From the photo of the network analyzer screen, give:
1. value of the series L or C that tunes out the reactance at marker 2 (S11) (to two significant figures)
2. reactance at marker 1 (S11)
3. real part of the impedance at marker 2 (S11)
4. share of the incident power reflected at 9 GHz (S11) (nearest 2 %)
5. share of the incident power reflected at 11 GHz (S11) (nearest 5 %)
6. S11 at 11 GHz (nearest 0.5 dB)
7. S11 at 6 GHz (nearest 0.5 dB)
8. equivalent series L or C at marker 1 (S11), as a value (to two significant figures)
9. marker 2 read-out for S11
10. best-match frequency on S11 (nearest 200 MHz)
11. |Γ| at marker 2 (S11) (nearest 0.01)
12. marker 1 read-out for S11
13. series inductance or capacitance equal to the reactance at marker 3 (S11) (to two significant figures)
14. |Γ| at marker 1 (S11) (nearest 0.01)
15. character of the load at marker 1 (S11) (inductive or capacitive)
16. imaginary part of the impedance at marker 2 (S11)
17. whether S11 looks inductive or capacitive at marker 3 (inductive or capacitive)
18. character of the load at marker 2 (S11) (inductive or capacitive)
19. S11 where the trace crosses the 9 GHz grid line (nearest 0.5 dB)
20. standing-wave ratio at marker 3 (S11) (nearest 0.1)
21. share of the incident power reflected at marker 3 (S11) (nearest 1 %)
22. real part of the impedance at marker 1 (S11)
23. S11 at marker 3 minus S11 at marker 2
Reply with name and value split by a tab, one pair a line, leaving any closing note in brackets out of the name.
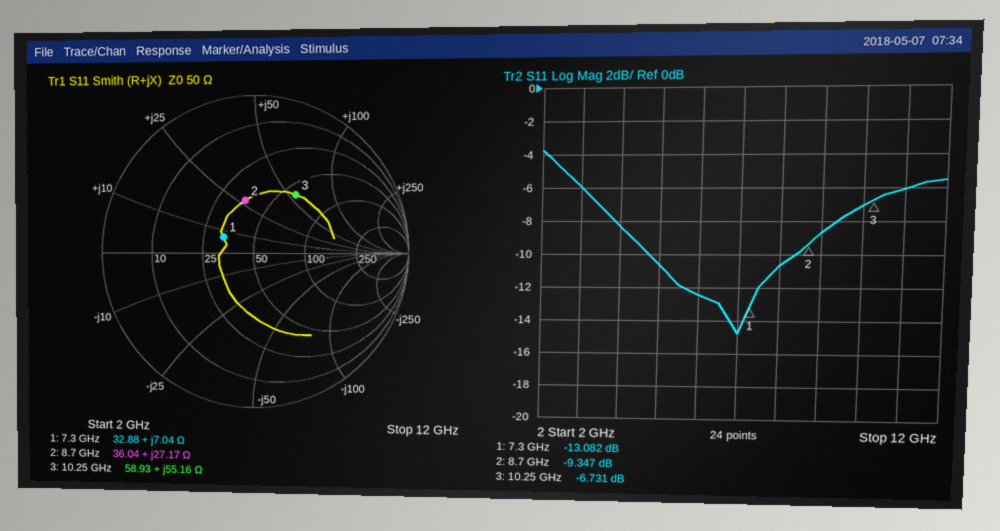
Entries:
value of the series L or C that tunes out the reactance at marker 2 (S11)	670 fF
reactance at marker 1	+7.04 Ω
real part of the impedance at marker 2	36.04 Ω
share of the incident power reflected at 9 GHz (S11)	14 %
share of the incident power reflected at 11 GHz (S11)	25 %
S11 at 11 GHz	-6.0 dB
S11 at 6 GHz	-12.5 dB
equivalent series L or C at marker 1 (S11), as a value	150 pH
marker 2 read-out for S11	-9.347 dB
best-match frequency on S11	7.0 GHz
|Γ| at marker 2 (S11)	0.34
marker 1 read-out for S11	-13.082 dB
series inductance or capacitance equal to the reactance at marker 3 (S11)	860 pH
|Γ| at marker 1 (S11)	0.22
character of the load at marker 1 (S11)	inductive
imaginary part of the impedance at marker 2	+27.17 Ω
whether S11 looks inductive or capacitive at marker 3	inductive
character of the load at marker 2 (S11)	inductive
S11 where the trace crosses the 9 GHz grid line	-8.5 dB
standing-wave ratio at marker 3 (S11)	2.7
share of the incident power reflected at marker 3 (S11)	21 %
real part of the impedance at marker 1	32.88 Ω
S11 at marker 3 minus S11 at marker 2	2.616 dB
